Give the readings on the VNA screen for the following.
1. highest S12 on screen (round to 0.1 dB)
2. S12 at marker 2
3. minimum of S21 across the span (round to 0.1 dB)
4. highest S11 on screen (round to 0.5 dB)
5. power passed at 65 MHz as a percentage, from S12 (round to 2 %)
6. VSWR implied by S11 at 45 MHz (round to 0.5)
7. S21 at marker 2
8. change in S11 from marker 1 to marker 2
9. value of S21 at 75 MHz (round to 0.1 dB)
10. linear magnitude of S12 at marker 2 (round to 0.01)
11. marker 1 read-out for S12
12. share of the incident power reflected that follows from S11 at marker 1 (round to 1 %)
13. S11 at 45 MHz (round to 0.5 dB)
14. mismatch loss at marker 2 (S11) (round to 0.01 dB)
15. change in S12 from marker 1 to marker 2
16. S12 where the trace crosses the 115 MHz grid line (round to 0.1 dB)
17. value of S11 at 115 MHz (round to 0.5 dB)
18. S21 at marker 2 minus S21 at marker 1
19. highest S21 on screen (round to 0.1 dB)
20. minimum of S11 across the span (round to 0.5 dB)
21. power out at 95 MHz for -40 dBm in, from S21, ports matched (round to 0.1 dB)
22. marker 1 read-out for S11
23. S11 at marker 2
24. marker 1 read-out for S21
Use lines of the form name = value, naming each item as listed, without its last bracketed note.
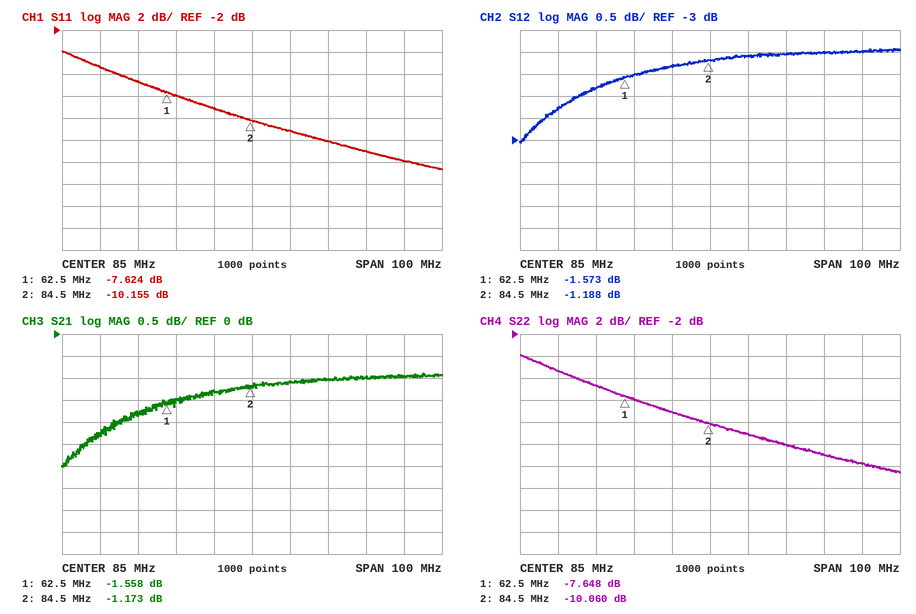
highest S12 on screen = -0.9 dB
S12 at marker 2 = -1.188 dB
minimum of S21 across the span = -3.0 dB
highest S11 on screen = -4.0 dB
power passed at 65 MHz as a percentage, from S12 = 70 %
VSWR implied by S11 at 45 MHz = 3.5
S21 at marker 2 = -1.173 dB
change in S11 from marker 1 to marker 2 = -2.531 dB
value of S21 at 75 MHz = -1.3 dB
linear magnitude of S12 at marker 2 = 0.87
marker 1 read-out for S12 = -1.573 dB
share of the incident power reflected that follows from S11 at marker 1 = 17 %
S11 at 45 MHz = -5.5 dB
mismatch loss at marker 2 (S11) = 0.44 dB
change in S12 from marker 1 to marker 2 = 0.385 dB
S12 where the trace crosses the 115 MHz grid line = -1.0 dB
value of S11 at 115 MHz = -13.0 dB
S21 at marker 2 minus S21 at marker 1 = 0.385 dB
highest S21 on screen = -0.9 dB
minimum of S11 across the span = -14.5 dB
power out at 95 MHz for -40 dBm in, from S21, ports matched = -41.1 dBm
marker 1 read-out for S11 = -7.624 dB
S11 at marker 2 = -10.155 dB
marker 1 read-out for S21 = -1.558 dB
